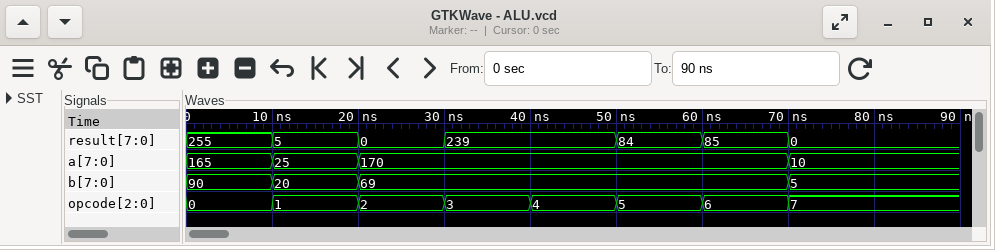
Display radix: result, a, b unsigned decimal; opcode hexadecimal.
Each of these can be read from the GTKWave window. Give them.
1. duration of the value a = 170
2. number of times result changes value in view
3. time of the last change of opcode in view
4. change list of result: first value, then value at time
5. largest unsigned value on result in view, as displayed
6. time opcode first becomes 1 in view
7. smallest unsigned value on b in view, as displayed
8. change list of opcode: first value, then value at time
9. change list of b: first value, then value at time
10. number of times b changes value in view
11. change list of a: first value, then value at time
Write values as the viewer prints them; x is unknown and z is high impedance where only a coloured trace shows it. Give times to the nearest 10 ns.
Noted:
50 ns
6
70 ns
255, 5 at 10 ns, 0 at 20 ns, 239 at 30 ns, 84 at 50 ns, 85 at 60 ns, 0 at 70 ns
255
10 ns
5
0, 1 at 10 ns, 2 at 20 ns, 3 at 30 ns, 4 at 40 ns, 5 at 50 ns, 6 at 60 ns, 7 at 70 ns
90, 20 at 10 ns, 69 at 20 ns, 5 at 70 ns
3
165, 25 at 10 ns, 170 at 20 ns, 10 at 70 ns
